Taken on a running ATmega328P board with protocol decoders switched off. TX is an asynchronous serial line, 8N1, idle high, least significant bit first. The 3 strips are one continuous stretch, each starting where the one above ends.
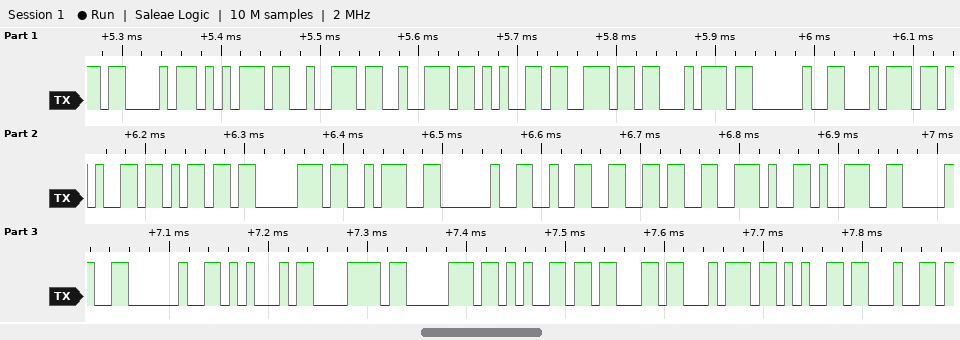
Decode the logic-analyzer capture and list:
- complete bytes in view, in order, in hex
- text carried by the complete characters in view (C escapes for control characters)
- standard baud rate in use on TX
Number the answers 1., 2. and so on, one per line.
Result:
1. 43 75 72 72 65 6E 74 20 74 65 6D 70 3A 20 32 36 2E 39 30 20 45 78 70 65 63 74 65 64
2. "Current temp: 26.90 Expected"
3. 115200 baud
